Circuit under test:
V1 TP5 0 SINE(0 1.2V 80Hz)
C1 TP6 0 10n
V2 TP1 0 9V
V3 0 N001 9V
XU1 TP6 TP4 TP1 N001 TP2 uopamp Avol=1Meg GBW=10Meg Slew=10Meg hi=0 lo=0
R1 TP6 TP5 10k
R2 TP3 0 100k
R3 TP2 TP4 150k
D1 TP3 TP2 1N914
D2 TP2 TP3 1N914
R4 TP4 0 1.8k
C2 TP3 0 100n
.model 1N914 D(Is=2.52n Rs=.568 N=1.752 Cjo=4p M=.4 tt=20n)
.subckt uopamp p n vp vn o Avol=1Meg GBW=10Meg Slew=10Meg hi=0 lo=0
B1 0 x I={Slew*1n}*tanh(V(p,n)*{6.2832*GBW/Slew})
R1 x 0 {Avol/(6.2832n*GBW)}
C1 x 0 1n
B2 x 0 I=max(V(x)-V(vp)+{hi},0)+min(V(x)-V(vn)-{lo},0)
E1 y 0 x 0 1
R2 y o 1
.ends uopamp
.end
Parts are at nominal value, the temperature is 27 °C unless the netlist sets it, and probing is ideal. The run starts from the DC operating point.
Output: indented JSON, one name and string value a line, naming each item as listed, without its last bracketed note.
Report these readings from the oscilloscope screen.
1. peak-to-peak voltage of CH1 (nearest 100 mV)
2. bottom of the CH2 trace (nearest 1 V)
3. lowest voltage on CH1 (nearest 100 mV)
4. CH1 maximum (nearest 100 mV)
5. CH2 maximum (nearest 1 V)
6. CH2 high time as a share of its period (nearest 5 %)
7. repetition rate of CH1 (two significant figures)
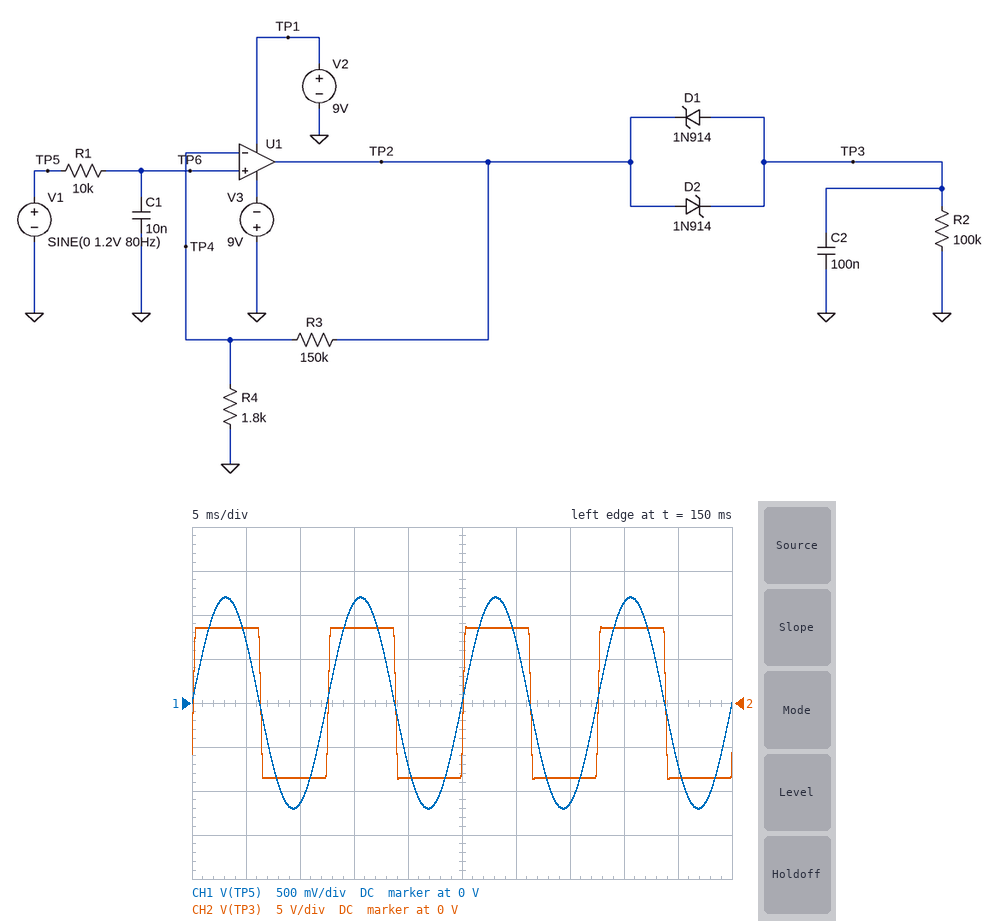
{
  "peak-to-peak voltage of CH1": "2.4 V",
  "bottom of the CH2 trace": "-9 V",
  "lowest voltage on CH1": "-1.2 V",
  "CH1 maximum": "1.2 V",
  "CH2 maximum": "9 V",
  "CH2 high time as a share of its period": "50 %",
  "repetition rate of CH1": "80 Hz"
}
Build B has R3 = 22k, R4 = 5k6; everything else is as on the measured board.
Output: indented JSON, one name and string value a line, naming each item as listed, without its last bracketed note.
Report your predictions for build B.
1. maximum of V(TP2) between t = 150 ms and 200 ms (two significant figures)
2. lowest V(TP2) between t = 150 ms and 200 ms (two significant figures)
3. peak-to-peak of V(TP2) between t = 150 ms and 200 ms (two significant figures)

{
  "maximum of V(TP2) between t = 150 ms and 200 ms": "5.9 V",
  "lowest V(TP2) between t = 150 ms and 200 ms": "-5.9 V",
  "peak-to-peak of V(TP2) between t = 150 ms and 200 ms": "12 V"
}
